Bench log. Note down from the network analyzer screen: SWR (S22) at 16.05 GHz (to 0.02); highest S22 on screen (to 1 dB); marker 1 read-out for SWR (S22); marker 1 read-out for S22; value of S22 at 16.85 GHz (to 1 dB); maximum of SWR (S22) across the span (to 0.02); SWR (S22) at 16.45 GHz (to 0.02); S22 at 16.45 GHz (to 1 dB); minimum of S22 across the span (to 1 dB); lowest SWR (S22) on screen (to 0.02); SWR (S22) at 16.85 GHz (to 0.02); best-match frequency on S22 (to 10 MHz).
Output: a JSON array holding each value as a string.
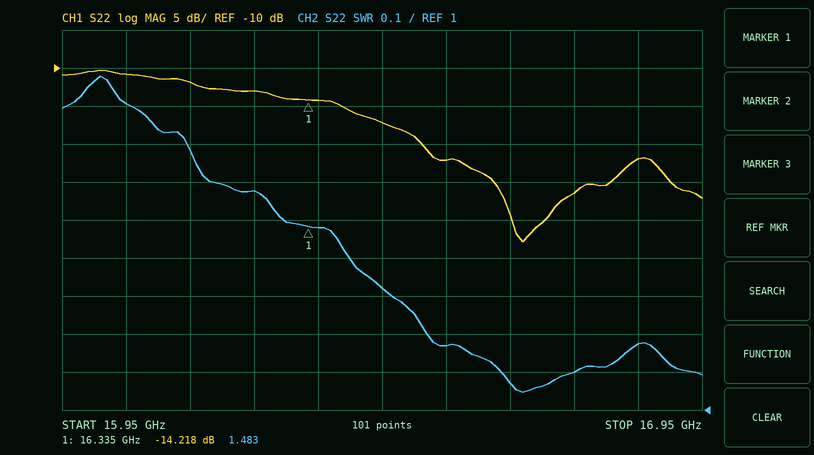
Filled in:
["1.80", "-10 dB", "1.483", "-14.218 dB", "-22 dB", "1.88", "1.32", "-17 dB", "-33 dB", "1.04", "1.18", "16.67 GHz"]
